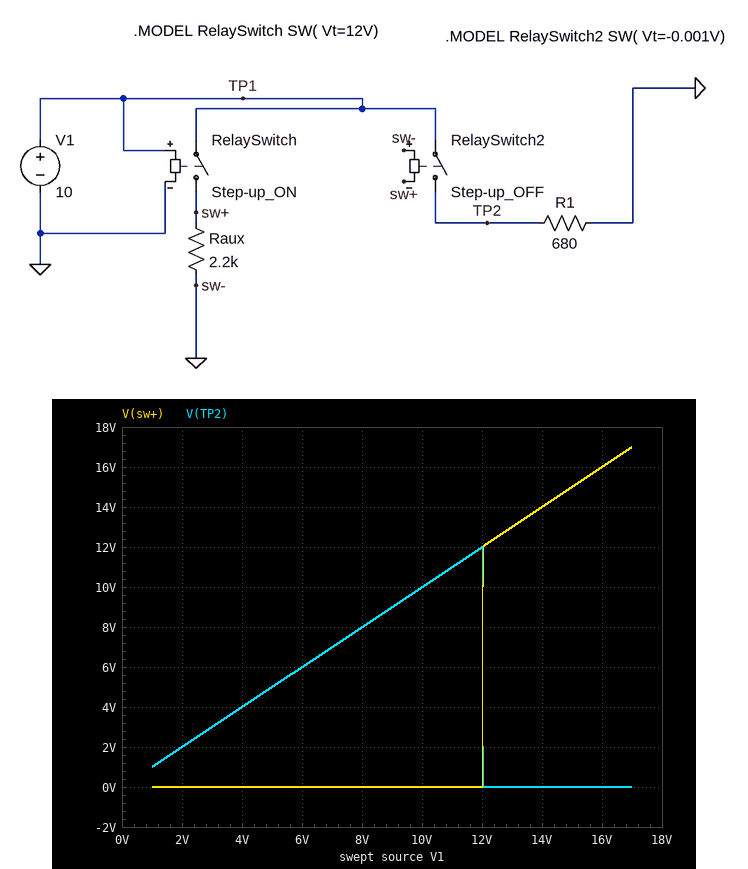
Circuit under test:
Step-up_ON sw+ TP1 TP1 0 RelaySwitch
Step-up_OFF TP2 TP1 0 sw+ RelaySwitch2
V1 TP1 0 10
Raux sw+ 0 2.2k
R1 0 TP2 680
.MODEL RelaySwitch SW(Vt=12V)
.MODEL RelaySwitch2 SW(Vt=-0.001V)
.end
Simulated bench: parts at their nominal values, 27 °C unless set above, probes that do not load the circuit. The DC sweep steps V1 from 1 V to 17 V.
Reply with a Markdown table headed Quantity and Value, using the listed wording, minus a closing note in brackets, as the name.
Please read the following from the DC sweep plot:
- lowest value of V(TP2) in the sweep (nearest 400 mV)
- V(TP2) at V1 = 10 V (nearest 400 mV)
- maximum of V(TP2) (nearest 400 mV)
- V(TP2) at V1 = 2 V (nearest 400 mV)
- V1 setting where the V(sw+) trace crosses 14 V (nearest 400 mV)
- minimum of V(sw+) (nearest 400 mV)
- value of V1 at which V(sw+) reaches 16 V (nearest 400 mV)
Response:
| Quantity | Value |
|---|---|
| lowest value of V(TP2) in the sweep | 0 V |
| V(TP2) at V1 = 10 V | 10.0 V |
| maximum of V(TP2) | 12.0 V |
| V(TP2) at V1 = 2 V | 2.0 V |
| V1 setting where the V(sw+) trace crosses 14 V | 14.0 V |
| minimum of V(sw+) | 0 V |
| value of V1 at which V(sw+) reaches 16 V | 16.0 V |
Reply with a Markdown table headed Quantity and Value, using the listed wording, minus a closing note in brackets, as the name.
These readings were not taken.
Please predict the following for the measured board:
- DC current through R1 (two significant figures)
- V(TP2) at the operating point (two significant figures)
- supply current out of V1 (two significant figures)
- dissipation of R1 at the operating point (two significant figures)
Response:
| Quantity | Value |
|---|---|
| DC current through R1 | 15 mA |
| V(TP2) at the operating point | 10 V |
| supply current out of V1 | 15 mA |
| dissipation of R1 at the operating point | 150 mW |
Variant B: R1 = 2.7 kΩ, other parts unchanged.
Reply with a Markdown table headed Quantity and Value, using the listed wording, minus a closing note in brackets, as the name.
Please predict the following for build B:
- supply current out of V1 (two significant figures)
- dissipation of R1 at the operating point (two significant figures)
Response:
| Quantity | Value |
|---|---|
| supply current out of V1 | 3.7 mA |
| dissipation of R1 at the operating point | 37 mW |
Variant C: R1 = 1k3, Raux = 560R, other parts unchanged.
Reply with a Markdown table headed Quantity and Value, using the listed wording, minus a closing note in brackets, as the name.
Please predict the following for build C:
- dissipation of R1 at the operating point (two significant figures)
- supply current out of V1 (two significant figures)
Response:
| Quantity | Value |
|---|---|
| dissipation of R1 at the operating point | 77 mW |
| supply current out of V1 | 7.7 mA |
